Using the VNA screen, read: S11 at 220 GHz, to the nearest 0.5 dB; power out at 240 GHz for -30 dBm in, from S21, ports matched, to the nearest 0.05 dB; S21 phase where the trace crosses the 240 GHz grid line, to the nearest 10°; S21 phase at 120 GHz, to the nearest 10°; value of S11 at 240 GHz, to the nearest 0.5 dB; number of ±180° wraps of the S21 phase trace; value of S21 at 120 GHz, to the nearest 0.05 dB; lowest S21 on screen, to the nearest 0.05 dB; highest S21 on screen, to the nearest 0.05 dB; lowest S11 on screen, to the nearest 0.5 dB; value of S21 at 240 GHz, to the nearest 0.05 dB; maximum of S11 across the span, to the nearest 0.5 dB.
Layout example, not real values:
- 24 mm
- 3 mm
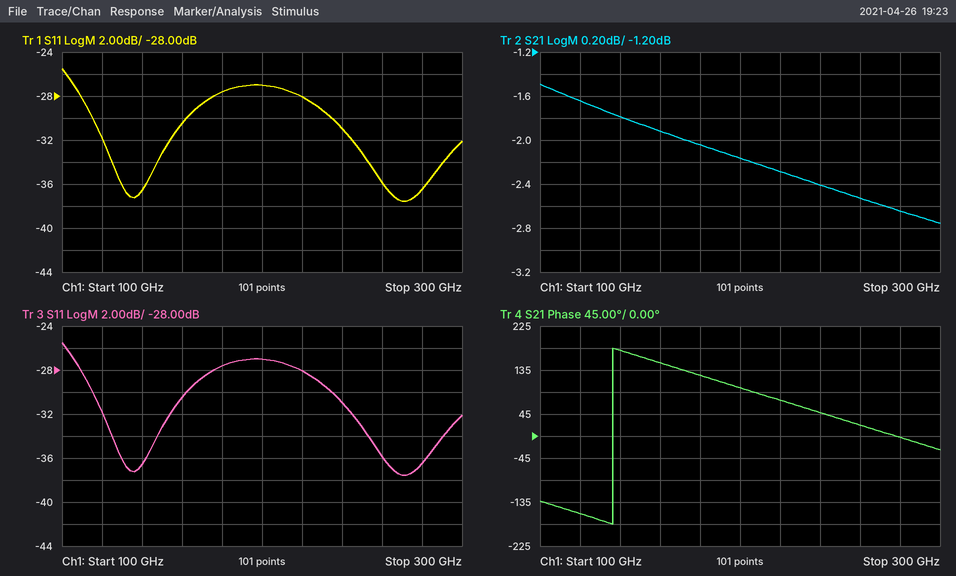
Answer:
- -28.0 dB
- -32.40 dBm
- 50°
- -160°
- -31.0 dB
- 1
- -1.65 dB
- -2.75 dB
- -1.50 dB
- -37.5 dB
- -2.40 dB
- -25.5 dB
